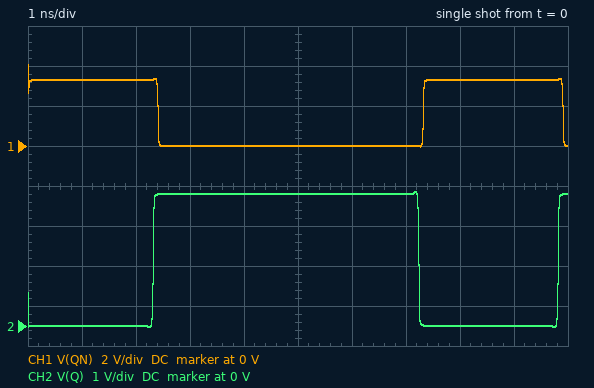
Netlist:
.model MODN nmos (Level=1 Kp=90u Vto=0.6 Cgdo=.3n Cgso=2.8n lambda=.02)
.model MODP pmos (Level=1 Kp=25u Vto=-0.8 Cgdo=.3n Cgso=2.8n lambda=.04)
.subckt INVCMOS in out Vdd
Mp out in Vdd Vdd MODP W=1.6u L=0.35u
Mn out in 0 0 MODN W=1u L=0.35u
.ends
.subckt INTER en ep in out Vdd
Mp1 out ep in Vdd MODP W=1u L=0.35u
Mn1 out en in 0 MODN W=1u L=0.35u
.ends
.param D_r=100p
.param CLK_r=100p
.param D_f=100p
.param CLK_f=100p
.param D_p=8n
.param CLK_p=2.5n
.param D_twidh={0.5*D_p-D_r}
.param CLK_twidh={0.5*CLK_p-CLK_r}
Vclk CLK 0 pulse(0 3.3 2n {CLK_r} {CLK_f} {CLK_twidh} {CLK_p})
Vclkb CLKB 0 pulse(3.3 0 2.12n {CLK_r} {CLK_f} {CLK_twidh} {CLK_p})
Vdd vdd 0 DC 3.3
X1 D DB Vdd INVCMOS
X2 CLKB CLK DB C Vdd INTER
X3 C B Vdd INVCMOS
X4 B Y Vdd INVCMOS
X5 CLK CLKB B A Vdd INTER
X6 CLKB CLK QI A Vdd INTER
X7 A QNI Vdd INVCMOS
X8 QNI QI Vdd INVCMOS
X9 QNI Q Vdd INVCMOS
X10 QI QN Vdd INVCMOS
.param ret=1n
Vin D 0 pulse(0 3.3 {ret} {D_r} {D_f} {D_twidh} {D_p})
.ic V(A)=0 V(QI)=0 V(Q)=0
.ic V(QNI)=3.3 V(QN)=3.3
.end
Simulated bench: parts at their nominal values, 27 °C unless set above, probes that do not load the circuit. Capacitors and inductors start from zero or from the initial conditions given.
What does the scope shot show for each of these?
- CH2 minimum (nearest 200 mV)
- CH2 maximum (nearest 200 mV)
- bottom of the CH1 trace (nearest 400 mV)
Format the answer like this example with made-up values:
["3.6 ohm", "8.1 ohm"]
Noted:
["0 V", "3.4 V", "0 V"]
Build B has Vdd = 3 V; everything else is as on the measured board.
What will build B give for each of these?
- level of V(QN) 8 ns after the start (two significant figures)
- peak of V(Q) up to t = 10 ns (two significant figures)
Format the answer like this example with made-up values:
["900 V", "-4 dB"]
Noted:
["3.0 V", "3.1 V"]
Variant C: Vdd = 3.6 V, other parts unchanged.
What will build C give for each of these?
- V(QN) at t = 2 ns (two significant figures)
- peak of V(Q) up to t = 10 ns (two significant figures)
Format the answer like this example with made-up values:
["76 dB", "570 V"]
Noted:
["3.6 V", "3.7 V"]
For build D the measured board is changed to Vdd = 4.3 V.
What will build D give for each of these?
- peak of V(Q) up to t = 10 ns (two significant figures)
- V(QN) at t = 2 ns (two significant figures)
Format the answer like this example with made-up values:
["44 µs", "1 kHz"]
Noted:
["4.4 V", "4.3 V"]
